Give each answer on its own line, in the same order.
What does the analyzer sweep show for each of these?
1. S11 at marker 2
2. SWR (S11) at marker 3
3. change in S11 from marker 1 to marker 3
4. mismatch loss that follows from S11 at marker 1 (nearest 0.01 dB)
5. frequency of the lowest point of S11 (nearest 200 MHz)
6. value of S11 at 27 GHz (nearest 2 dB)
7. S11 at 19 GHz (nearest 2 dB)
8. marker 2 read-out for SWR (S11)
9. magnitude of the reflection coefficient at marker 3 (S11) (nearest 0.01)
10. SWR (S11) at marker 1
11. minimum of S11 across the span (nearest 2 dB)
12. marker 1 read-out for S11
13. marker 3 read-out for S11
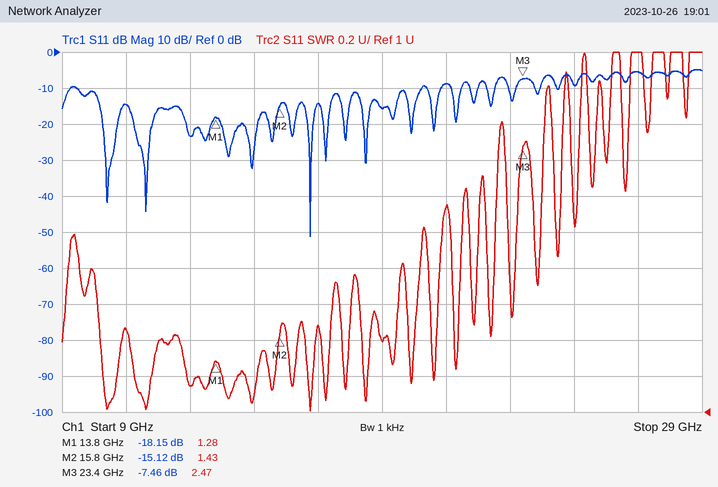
-15.12 dB
2.47
10.69 dB
0.07 dB
16.8 GHz
-6 dB
-16 dB
1.43
0.42
1.28
-52 dB
-18.15 dB
-7.46 dB
